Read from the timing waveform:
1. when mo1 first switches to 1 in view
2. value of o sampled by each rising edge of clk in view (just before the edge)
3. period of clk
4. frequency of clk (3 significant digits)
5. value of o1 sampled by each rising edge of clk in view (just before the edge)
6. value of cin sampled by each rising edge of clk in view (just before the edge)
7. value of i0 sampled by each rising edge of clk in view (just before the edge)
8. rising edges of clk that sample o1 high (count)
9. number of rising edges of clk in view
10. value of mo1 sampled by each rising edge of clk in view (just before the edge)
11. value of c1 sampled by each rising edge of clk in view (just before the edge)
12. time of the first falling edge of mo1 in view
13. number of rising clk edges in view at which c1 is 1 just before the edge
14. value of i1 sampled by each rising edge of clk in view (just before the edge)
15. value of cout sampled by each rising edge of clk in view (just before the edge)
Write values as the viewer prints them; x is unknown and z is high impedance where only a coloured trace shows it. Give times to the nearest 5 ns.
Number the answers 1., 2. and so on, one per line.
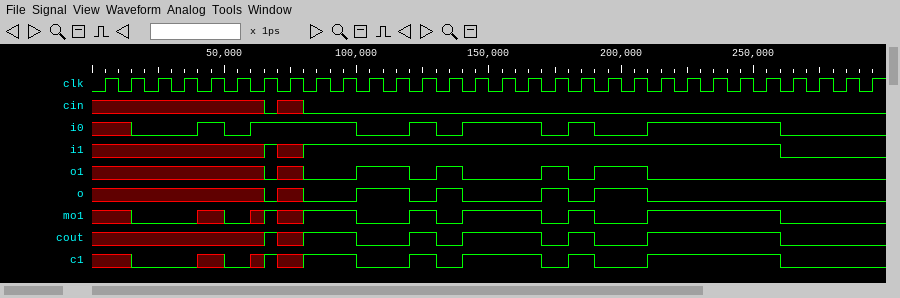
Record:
1. 65 ns
2. x x x x x x x x 0 0 1 1 0 1 0 0 0 1 0 1 1 0 0 0 0 0 0 0 0 0
3. 10 ns
4. 100 MHz
5. x x x x x x x x 0 0 1 1 0 1 0 0 0 1 0 1 1 0 0 0 0 0 0 0 0 0
6. x x x x x x x x 0 0 0 0 0 0 0 0 0 0 0 0 0 0 0 0 0 0 0 0 0 0
7. x x 0 0 1 0 1 1 1 1 0 0 1 0 1 1 1 0 1 0 0 1 1 1 1 1 0 0 0 0
8. 6
9. 30
10. x x 0 0 x 0 x x 1 1 0 0 1 0 1 1 1 0 1 0 0 1 1 1 1 1 0 0 0 0
11. x x 0 0 x 0 x x 1 1 0 0 1 0 1 1 1 0 1 0 0 1 1 1 1 1 0 0 0 0
12. 100 ns
13. 12
14. x x x x x x x x 1 1 1 1 1 1 1 1 1 1 1 1 1 1 1 1 1 1 0 0 0 0
15. x x x x x x x x 1 1 0 0 1 0 1 1 1 0 1 0 0 1 1 1 1 1 0 0 0 0
